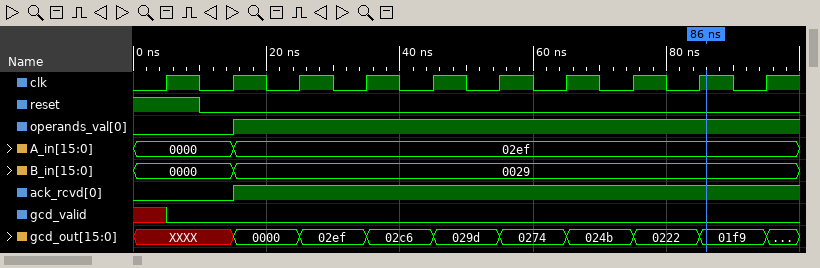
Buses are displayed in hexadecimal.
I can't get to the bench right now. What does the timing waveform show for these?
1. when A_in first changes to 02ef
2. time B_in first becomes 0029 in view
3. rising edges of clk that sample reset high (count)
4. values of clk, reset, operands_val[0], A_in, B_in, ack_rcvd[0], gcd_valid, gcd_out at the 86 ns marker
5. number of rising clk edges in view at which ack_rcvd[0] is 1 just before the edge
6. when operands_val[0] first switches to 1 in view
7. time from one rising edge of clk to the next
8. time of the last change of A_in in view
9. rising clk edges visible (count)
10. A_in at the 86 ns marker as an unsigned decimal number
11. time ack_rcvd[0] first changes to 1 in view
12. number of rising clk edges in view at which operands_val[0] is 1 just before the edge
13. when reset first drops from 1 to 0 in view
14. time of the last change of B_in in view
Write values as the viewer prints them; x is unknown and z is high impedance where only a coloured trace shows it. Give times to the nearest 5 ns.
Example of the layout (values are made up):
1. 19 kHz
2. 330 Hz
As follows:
1. 15 ns
2. 15 ns
3. 1
4. clk=1, reset=0, operands_val[0]=1, A_in=02ef, B_in=0029, ack_rcvd[0]=1, gcd_valid=0, gcd_out=01f9
5. 8
6. 15 ns
7. 10 ns
8. 15 ns
9. 10
10. 751
11. 15 ns
12. 8
13. 10 ns
14. 15 ns
